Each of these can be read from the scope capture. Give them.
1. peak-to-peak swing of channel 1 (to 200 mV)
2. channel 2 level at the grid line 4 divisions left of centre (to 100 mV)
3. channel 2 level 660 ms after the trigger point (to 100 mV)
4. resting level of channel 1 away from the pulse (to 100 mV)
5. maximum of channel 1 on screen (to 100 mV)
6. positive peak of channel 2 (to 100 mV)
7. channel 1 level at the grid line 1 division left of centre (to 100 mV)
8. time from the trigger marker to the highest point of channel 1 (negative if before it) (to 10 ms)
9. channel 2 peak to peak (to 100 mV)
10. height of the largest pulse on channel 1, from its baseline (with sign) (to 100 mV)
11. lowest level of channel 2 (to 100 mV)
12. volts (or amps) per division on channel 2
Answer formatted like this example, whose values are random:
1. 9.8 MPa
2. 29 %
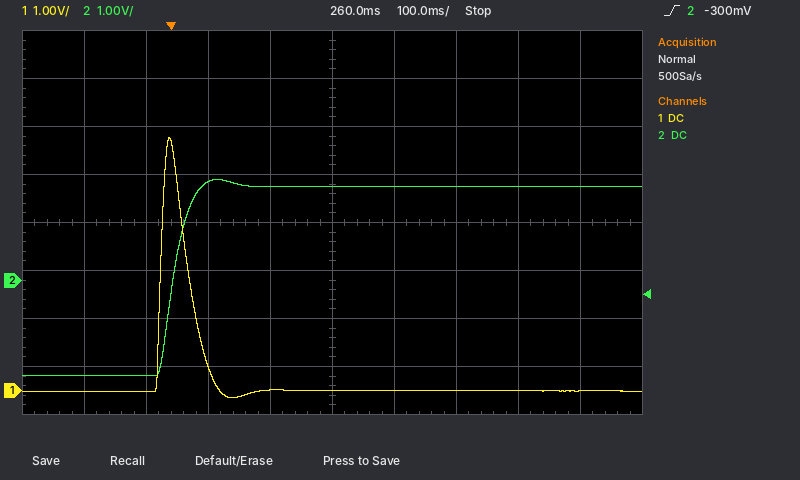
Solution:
1. 5.4 V
2. -2.0 V
3. 2.0 V
4. 0.0 V
5. 5.3 V
6. 2.1 V
7. 0.0 V
8. 0 ms
9. 4.1 V
10. +5.3 V
11. -2.0 V
12. 1 V
